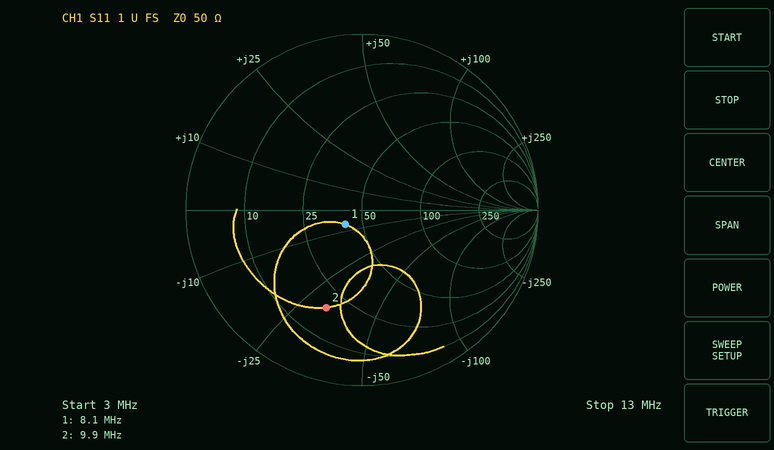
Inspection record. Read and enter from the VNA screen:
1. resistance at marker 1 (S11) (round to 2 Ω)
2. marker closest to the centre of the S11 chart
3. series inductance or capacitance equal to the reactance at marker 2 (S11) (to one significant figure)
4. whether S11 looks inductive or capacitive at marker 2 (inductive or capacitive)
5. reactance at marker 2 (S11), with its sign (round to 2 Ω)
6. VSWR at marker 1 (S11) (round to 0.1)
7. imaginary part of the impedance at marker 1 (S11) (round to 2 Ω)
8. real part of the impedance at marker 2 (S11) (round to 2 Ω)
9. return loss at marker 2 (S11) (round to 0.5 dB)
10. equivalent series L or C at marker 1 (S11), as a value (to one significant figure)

40 Ω
marker 1
500 pF
capacitive
-32 Ω
1.3
-6 Ω
18 Ω
4.5 dB
3 nF
